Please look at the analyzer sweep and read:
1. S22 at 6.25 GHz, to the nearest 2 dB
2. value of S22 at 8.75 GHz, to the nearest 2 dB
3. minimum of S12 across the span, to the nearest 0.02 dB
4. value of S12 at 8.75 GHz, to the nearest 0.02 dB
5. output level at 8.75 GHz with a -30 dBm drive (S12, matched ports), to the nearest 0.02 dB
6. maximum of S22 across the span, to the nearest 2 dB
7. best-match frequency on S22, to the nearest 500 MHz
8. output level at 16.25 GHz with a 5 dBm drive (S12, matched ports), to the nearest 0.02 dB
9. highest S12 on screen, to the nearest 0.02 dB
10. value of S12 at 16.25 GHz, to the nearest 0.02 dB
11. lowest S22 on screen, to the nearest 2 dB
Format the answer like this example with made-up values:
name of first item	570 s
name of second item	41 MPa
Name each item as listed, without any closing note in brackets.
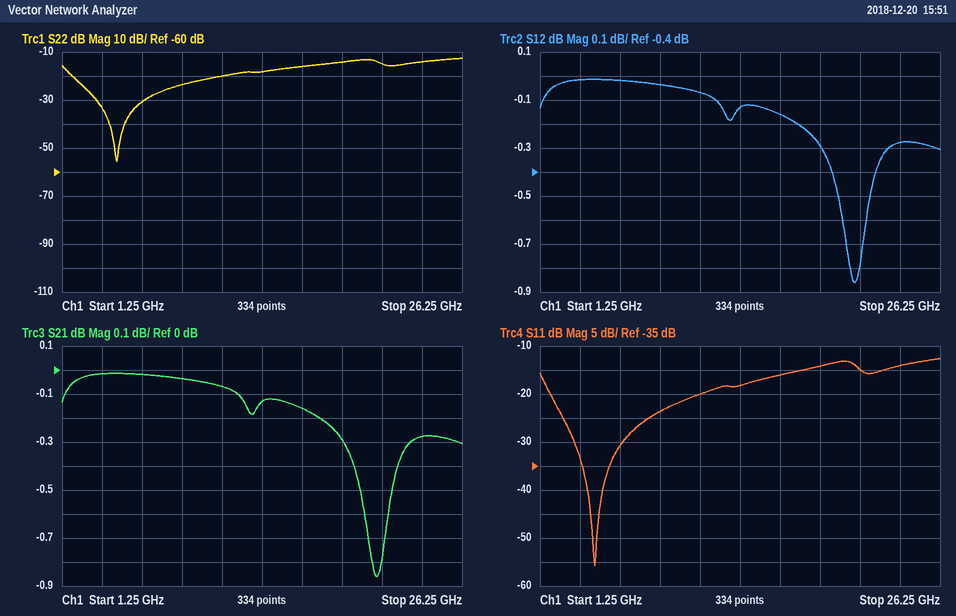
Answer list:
S22 at 6.25 GHz, to the nearest 2 dB	-30 dB
value of S22 at 8.75 GHz, to the nearest 2 dB	-24 dB
minimum of S12 across the span, to the nearest 0.02 dB	-0.86 dB
value of S12 at 8.75 GHz, to the nearest 0.02 dB	-0.04 dB
output level at 8.75 GHz with a -30 dBm drive (S12, matched ports), to the nearest 0.02 dB	-30.04 dBm
maximum of S22 across the span, to the nearest 2 dB	-12 dB
best-match frequency on S22, to the nearest 500 MHz	4.5 GHz
output level at 16.25 GHz with a 5 dBm drive (S12, matched ports), to the nearest 0.02 dB	4.84 dBm
highest S12 on screen, to the nearest 0.02 dB	-0.02 dB
value of S12 at 16.25 GHz, to the nearest 0.02 dB	-0.16 dB
lowest S22 on screen, to the nearest 2 dB	-56 dB
